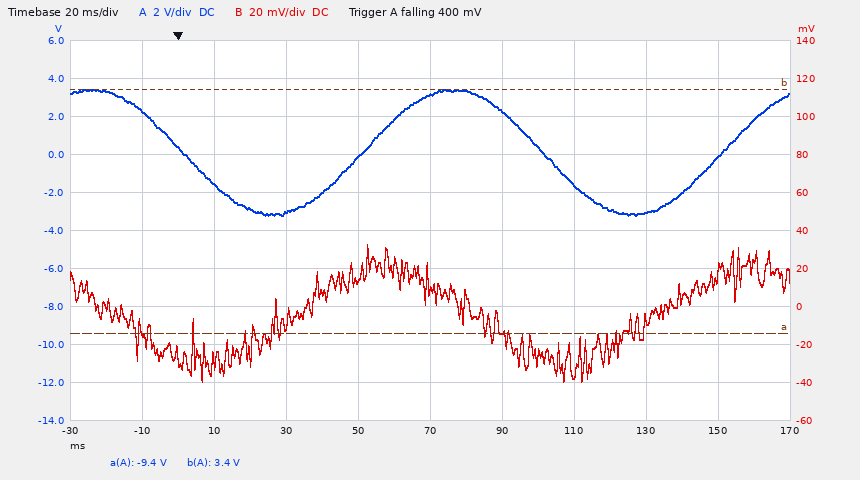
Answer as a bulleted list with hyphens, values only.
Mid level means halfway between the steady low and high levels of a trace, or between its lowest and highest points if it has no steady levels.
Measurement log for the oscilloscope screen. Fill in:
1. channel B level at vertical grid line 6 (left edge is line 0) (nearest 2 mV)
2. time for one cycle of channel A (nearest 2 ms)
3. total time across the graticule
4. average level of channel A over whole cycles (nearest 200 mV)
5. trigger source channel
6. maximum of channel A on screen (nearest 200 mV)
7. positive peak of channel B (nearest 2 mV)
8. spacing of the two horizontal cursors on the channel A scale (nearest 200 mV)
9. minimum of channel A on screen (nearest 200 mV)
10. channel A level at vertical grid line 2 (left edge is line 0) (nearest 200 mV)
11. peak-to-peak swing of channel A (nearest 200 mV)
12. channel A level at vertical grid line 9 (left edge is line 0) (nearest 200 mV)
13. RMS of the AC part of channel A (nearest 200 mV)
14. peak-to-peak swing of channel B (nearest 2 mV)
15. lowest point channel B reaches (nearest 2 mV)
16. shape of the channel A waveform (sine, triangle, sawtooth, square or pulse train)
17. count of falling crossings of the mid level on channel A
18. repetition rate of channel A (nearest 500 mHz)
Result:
- -14 mV
- 100 ms
- 200 ms
- 200 mV
- channel A
- 3.4 V
- 32 mV
- 12.8 V
- -3.2 V
- -1.6 V
- 6.6 V
- -200 mV
- 2.4 V
- 72 mV
- -40 mV
- sine
- 2
- 10.0 Hz
